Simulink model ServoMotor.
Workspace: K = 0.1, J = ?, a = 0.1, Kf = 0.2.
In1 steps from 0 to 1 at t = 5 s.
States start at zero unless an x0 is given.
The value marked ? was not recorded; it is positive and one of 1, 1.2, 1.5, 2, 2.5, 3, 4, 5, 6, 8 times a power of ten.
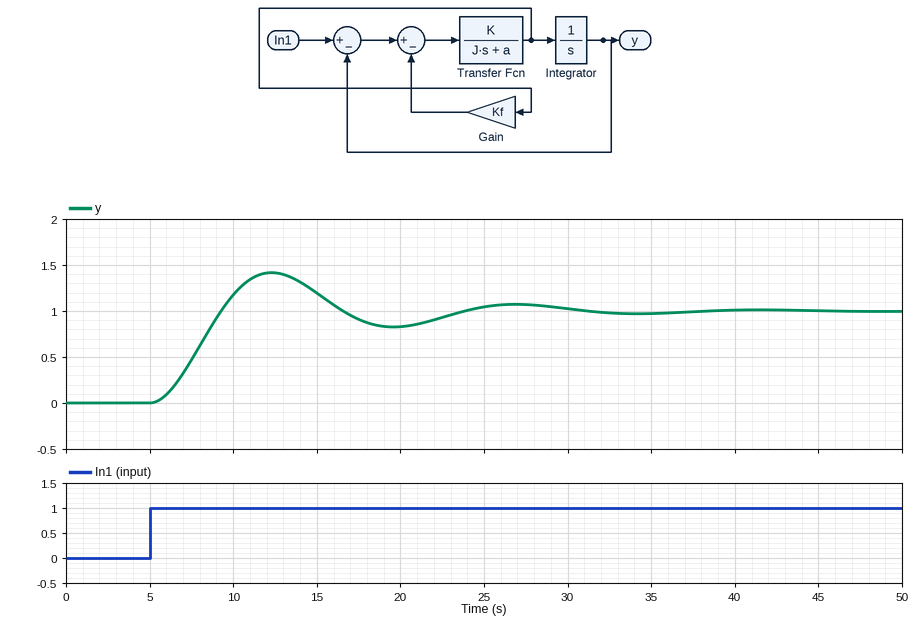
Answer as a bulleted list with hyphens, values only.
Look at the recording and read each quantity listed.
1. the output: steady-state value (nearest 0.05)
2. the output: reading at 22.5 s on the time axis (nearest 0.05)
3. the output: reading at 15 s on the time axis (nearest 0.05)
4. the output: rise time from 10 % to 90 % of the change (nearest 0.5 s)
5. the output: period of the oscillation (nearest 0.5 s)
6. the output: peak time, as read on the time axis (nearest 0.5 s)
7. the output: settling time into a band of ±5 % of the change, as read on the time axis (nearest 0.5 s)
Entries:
- 1.00
- 0.95
- 1.20
- 3.0 s
- 14.5 s
- 12.5 s
- 29.0 s
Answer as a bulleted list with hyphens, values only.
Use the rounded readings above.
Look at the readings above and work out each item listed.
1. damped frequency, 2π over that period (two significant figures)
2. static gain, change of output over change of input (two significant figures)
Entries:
- 0.43 rad/s
- 1.0
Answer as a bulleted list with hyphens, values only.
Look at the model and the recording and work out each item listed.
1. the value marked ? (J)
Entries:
- 0.5
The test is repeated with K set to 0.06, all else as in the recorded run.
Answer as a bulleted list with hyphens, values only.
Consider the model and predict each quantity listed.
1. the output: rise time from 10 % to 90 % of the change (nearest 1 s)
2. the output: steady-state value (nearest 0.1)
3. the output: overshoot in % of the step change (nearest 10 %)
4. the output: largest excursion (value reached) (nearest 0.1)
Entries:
- 4 s
- 1.0
- 30 %
- 1.3
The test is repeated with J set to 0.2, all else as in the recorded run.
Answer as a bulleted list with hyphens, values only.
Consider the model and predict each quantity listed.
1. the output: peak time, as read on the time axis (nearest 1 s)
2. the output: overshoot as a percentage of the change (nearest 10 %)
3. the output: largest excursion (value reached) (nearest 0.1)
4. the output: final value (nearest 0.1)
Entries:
- 10 s
- 20 %
- 1.2
- 1.0
